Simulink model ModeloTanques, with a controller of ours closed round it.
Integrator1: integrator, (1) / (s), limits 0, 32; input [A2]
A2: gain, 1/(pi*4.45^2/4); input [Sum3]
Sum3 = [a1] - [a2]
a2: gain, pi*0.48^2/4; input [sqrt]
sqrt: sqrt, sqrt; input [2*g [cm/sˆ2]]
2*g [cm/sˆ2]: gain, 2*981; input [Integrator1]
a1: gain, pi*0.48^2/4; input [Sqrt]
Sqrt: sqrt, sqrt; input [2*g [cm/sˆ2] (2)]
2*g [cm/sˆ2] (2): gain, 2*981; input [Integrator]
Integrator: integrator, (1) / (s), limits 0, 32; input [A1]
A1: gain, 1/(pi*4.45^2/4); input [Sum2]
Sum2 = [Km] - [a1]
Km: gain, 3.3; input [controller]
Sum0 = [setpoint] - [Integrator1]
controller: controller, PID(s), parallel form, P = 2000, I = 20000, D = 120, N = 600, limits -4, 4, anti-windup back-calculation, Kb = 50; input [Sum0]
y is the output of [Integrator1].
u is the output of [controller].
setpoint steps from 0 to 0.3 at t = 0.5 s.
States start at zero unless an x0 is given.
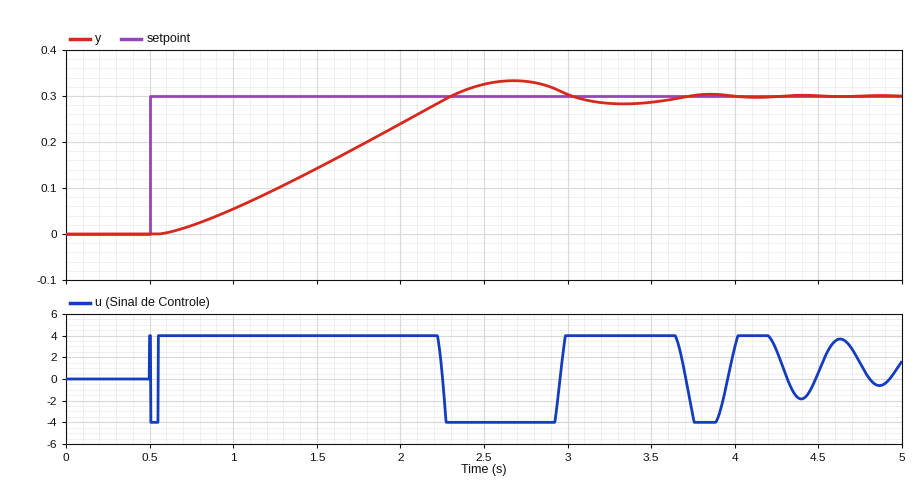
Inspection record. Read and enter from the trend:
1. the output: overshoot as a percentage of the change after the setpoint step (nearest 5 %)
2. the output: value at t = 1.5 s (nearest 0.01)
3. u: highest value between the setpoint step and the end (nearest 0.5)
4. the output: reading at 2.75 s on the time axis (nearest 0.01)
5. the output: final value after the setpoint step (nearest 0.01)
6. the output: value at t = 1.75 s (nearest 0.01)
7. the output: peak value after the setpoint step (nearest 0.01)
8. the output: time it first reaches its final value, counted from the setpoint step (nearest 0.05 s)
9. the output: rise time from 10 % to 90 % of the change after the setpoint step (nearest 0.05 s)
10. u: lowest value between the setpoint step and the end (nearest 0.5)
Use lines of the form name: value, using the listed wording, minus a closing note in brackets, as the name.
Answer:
the output: overshoot as a percentage of the change after the setpoint step: 10 %
the output: value at t = 1.5 s: 0.14
u: highest value between the setpoint step and the end: 4.0
the output: reading at 2.75 s on the time axis: 0.33
the output: final value after the setpoint step: 0.30
the output: value at t = 1.75 s: 0.19
the output: peak value after the setpoint step: 0.33
the output: time it first reaches its final value, counted from the setpoint step: 1.80 s
the output: rise time from 10 % to 90 % of the change after the setpoint step: 1.30 s
u: lowest value between the setpoint step and the end: -4.0
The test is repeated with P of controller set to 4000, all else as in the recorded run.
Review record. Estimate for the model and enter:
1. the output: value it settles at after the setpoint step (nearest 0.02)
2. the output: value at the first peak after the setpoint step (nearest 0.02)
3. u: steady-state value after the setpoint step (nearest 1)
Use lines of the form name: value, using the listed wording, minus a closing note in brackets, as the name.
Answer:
the output: value it settles at after the setpoint step: 0.30
the output: value at the first peak after the setpoint step: 0.32
u: steady-state value after the setpoint step: 1
